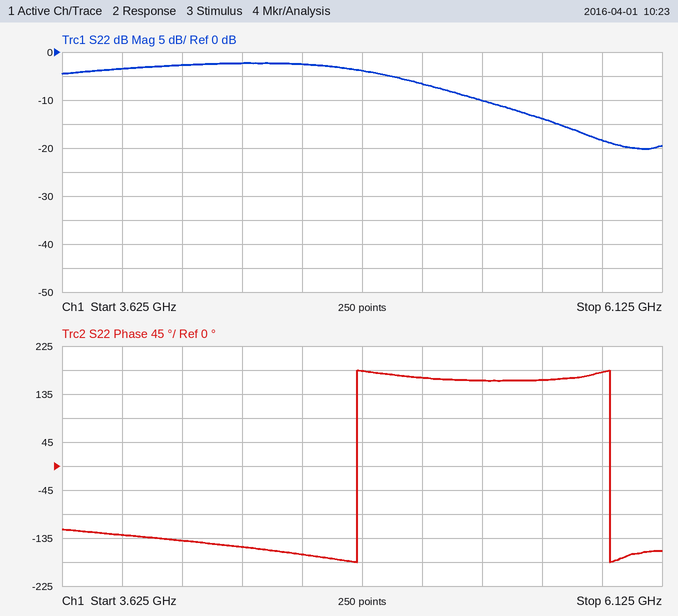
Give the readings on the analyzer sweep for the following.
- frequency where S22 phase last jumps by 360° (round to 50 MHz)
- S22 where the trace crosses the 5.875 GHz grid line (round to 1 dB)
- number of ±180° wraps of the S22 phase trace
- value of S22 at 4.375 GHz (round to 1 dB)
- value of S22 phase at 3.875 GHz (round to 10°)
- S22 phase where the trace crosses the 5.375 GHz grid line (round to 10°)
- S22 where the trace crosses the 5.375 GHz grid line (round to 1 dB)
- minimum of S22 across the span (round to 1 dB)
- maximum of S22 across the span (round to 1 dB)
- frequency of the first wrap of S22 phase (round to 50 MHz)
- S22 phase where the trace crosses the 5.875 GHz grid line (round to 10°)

5.90 GHz
-18 dB
2
-2 dB
-130°
160°
-10 dB
-20 dB
-2 dB
4.85 GHz
180°
